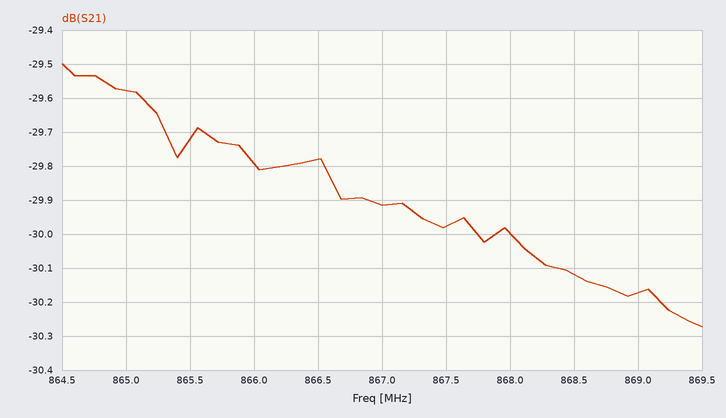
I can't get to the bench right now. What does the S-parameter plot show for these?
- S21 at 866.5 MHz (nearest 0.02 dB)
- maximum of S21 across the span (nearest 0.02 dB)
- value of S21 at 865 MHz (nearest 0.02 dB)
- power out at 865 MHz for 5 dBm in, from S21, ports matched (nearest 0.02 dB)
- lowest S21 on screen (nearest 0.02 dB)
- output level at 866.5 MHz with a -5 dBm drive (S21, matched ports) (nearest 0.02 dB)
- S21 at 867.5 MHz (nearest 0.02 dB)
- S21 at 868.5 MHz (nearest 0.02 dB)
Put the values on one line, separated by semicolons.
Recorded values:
-29.78 dB; -29.50 dB; -29.58 dB; -24.58 dBm; -30.28 dB; -34.78 dBm; -29.98 dB; -30.12 dB
